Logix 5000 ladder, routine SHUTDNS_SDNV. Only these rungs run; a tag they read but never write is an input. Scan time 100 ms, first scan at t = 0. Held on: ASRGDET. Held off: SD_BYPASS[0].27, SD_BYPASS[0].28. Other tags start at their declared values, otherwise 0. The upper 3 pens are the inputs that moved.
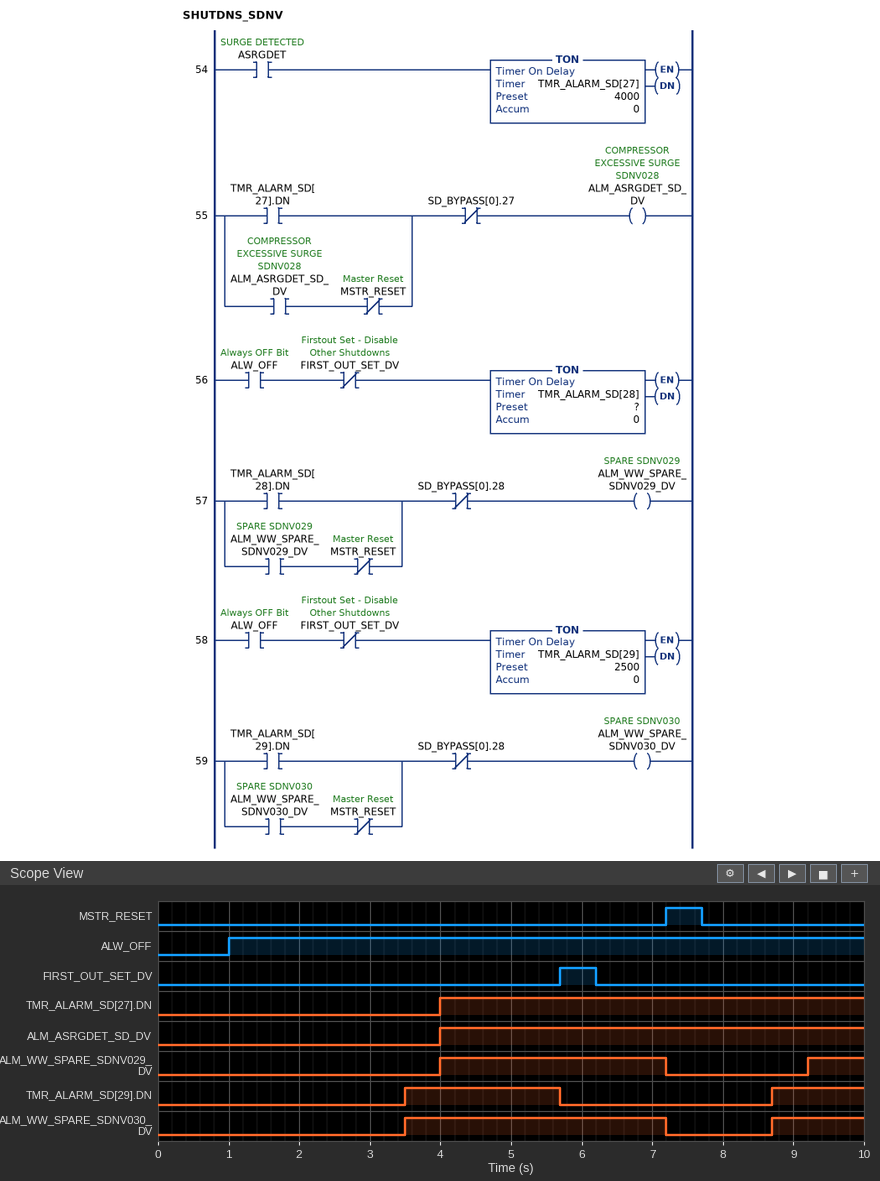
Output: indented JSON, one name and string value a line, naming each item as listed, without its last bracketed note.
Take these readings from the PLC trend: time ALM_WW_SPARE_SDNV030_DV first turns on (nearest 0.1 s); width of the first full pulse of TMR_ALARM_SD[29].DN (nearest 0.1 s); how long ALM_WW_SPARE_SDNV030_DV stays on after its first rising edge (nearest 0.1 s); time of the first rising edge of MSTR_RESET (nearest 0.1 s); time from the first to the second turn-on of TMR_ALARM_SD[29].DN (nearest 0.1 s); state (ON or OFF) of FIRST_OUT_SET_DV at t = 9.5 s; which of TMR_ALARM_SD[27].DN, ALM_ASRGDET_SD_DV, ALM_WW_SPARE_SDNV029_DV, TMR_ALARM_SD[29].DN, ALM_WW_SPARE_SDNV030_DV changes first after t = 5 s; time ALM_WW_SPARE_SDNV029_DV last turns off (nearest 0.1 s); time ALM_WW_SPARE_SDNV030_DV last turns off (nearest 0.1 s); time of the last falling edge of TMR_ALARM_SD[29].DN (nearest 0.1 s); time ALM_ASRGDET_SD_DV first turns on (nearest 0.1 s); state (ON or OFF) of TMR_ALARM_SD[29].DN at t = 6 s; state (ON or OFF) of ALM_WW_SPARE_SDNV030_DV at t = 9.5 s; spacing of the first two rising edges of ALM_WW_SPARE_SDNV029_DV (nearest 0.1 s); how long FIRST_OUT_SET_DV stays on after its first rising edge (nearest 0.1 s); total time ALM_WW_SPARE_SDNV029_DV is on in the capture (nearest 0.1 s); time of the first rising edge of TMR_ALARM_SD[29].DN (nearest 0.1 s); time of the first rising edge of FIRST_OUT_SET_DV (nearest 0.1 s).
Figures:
{
  "time ALM_WW_SPARE_SDNV030_DV first turns on": "3.5 s",
  "width of the first full pulse of TMR_ALARM_SD[29].DN": "2.2 s",
  "how long ALM_WW_SPARE_SDNV030_DV stays on after its first rising edge": "3.7 s",
  "time of the first rising edge of MSTR_RESET": "7.2 s",
  "time from the first to the second turn-on of TMR_ALARM_SD[29].DN": "5.2 s",
  "state (ON or OFF) of FIRST_OUT_SET_DV at t = 9.5 s": "OFF",
  "which of TMR_ALARM_SD[27].DN, ALM_ASRGDET_SD_DV, ALM_WW_SPARE_SDNV029_DV, TMR_ALARM_SD[29].DN, ALM_WW_SPARE_SDNV030_DV changes first after t = 5 s": "TMR_ALARM_SD[29].DN",
  "time ALM_WW_SPARE_SDNV029_DV last turns off": "7.2 s",
  "time ALM_WW_SPARE_SDNV030_DV last turns off": "7.2 s",
  "time of the last falling edge of TMR_ALARM_SD[29].DN": "5.7 s",
  "time ALM_ASRGDET_SD_DV first turns on": "4.0 s",
  "state (ON or OFF) of TMR_ALARM_SD[29].DN at t = 6 s": "OFF",
  "state (ON or OFF) of ALM_WW_SPARE_SDNV030_DV at t = 9.5 s": "ON",
  "spacing of the first two rising edges of ALM_WW_SPARE_SDNV029_DV": "5.2 s",
  "how long FIRST_OUT_SET_DV stays on after its first rising edge": "0.5 s",
  "total time ALM_WW_SPARE_SDNV029_DV is on in the capture": "4.0 s",
  "time of the first rising edge of TMR_ALARM_SD[29].DN": "3.5 s",
  "time of the first rising edge of FIRST_OUT_SET_DV": "5.7 s"
}
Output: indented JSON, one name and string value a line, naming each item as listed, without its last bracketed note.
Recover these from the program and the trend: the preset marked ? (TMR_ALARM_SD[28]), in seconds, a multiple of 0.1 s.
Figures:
{
  "the preset marked ? (TMR_ALARM_SD[28]), in seconds, a multiple of 0.1 s": "3.0 s"
}
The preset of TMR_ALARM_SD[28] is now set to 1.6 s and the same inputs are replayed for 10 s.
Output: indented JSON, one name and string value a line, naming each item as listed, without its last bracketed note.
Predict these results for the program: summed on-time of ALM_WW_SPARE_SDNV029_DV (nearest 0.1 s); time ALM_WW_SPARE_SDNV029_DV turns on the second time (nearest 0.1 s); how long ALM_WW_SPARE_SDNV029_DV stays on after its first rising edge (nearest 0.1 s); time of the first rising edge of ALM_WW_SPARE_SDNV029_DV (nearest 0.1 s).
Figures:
{
  "summed on-time of ALM_WW_SPARE_SDNV029_DV": "6.8 s",
  "time ALM_WW_SPARE_SDNV029_DV turns on the second time": "7.8 s",
  "how long ALM_WW_SPARE_SDNV029_DV stays on after its first rising edge": "4.6 s",
  "time of the first rising edge of ALM_WW_SPARE_SDNV029_DV": "2.6 s"
}
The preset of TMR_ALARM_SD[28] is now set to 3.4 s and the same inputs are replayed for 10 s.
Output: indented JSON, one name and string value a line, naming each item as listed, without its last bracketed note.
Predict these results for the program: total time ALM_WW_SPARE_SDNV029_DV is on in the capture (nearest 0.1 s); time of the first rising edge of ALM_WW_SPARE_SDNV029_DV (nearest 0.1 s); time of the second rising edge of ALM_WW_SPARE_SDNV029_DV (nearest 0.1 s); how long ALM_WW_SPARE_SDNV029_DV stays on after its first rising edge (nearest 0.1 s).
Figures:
{
  "total time ALM_WW_SPARE_SDNV029_DV is on in the capture": "3.2 s",
  "time of the first rising edge of ALM_WW_SPARE_SDNV029_DV": "4.4 s",
  "time of the second rising edge of ALM_WW_SPARE_SDNV029_DV": "9.6 s",
  "how long ALM_WW_SPARE_SDNV029_DV stays on after its first rising edge": "2.8 s"
}
